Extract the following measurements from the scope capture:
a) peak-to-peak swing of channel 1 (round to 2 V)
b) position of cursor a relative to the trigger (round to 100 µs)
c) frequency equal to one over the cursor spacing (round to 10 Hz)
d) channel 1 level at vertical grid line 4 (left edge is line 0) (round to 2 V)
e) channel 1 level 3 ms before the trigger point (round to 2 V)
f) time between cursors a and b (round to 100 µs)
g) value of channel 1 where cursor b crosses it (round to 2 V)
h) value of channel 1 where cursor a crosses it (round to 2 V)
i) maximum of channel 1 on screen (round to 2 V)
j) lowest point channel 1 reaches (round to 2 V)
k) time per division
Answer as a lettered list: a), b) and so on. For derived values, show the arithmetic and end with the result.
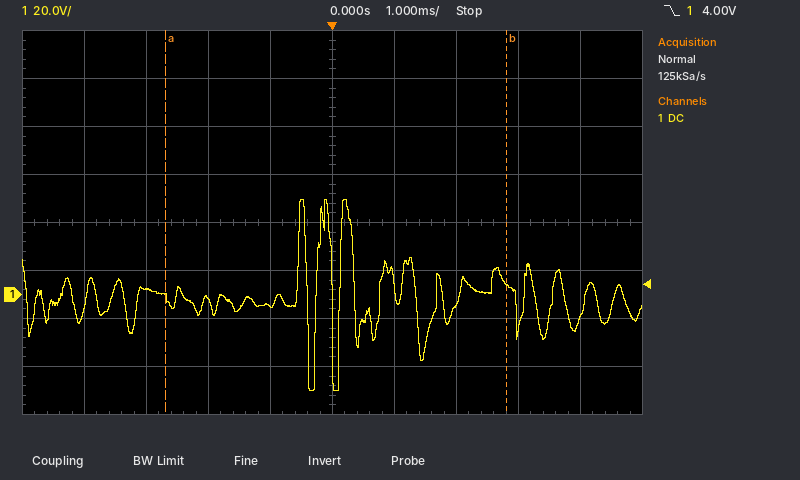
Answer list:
a) 40 V − (-40 V) = 80 V
b) -2.7 ms
c) 1 / 5.5 ms ≈ 180 Hz
d) -4 V
e) 2 V
f) 5.5 ms
g) 4 V
h) -2 V
i) 40 V
j) -40 V
k) 1 ms
